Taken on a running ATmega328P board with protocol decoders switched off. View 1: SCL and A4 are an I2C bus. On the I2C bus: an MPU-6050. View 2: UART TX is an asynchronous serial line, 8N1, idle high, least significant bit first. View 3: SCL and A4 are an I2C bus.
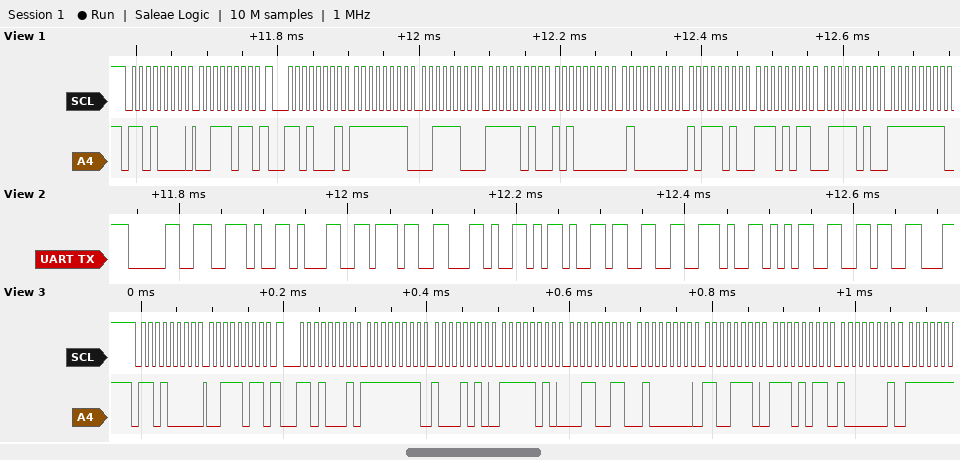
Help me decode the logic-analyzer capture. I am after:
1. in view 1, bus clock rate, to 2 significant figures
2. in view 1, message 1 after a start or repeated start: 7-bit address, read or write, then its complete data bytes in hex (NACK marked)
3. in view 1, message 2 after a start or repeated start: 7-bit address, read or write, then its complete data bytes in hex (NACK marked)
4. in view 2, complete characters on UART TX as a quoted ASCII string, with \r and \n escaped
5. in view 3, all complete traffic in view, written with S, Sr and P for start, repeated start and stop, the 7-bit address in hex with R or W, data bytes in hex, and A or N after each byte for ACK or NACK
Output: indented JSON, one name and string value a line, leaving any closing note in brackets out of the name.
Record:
{
  "in view 1, bus clock rate, to 2 significant figures": "100 kHz",
  "in view 1, message 1 after a start or repeated start: 7-bit address, read or write, then its complete data bytes in hex": "0x68 write: 3B",
  "in view 1, message 2 after a start or repeated start: 7-bit address, read or write, then its complete data bytes in hex": "0x68 read: FF 3C FA A0 40 BA EB 7A FF",
  "in view 2, complete characters on UART TX as a quoted ASCII string, with \\r and \\n escaped": "\"0.17,-3.56\"",
  "in view 3, all complete traffic in view, written with S, Sr and P for start, repeated start and stop, the 7-bit address in hex with R or W, data bytes in hex, and A or N after each byte for ACK or NACK": "S 68W A 3B A Sr 68R A FF A 8A A FA A 33 A 40 A CE A EB A 81 A"
}
